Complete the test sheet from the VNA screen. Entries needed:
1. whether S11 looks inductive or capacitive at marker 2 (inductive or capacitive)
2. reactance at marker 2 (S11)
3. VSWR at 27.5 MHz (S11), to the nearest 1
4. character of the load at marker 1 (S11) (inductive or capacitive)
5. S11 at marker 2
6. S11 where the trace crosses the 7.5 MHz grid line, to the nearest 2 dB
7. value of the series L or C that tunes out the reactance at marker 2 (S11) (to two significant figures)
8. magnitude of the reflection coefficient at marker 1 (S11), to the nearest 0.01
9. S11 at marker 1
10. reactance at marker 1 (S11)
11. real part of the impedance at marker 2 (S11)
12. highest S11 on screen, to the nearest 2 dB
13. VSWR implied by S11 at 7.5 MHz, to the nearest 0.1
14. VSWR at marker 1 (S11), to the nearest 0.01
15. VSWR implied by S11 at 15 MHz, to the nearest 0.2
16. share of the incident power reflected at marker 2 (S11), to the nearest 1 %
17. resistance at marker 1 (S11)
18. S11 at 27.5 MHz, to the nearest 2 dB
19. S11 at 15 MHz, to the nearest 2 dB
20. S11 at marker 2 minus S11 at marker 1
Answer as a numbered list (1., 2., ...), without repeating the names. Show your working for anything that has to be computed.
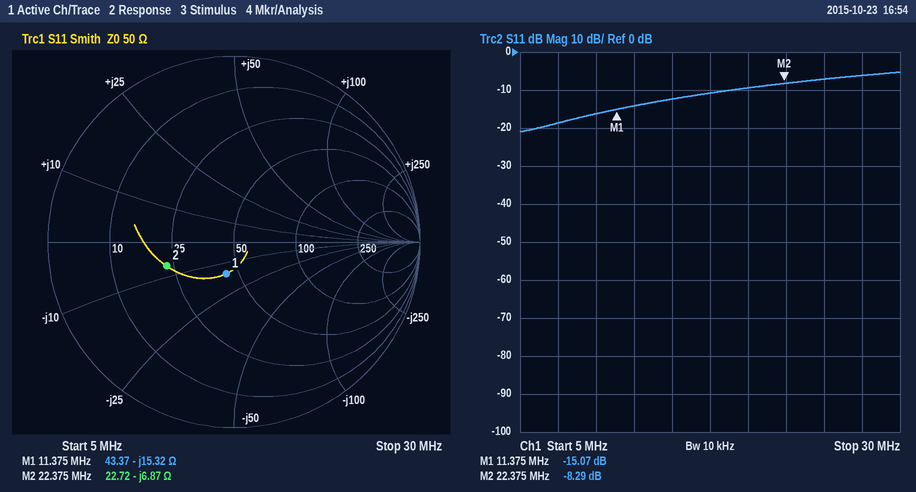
1. capacitive
2. -6.87 Ω
3. |Γ| = 10^(-6/20) = 0.5012; VSWR = (1 + 0.5012)/(1 − 0.5012) ≈ 3
4. capacitive
5. -8.29 dB
6. -18 dB
7. L = 6.87 Ω/(2π × 22.375 MHz) ≈ 49 nH
8. 10^(-15.07/20) ≈ 0.18
9. -15.07 dB
10. -15.32 Ω
11. 22.72 Ω
12. -6 dB
13. |Γ| = 10^(-18/20) = 0.1259; VSWR = (1 + 0.1259)/(1 − 0.1259) ≈ 1.3
14. 1.43
15. |Γ| = 10^(-12/20) = 0.2512; VSWR = (1 + 0.2512)/(1 − 0.2512) ≈ 1.67, so 1.6 to the nearest 0.2
16. 10^(-8.29/10) ≈ 15 %
17. 43.37 Ω
18. -6 dB
19. -12 dB
20. -8.29 − (-15.07) = 6.78 dB
